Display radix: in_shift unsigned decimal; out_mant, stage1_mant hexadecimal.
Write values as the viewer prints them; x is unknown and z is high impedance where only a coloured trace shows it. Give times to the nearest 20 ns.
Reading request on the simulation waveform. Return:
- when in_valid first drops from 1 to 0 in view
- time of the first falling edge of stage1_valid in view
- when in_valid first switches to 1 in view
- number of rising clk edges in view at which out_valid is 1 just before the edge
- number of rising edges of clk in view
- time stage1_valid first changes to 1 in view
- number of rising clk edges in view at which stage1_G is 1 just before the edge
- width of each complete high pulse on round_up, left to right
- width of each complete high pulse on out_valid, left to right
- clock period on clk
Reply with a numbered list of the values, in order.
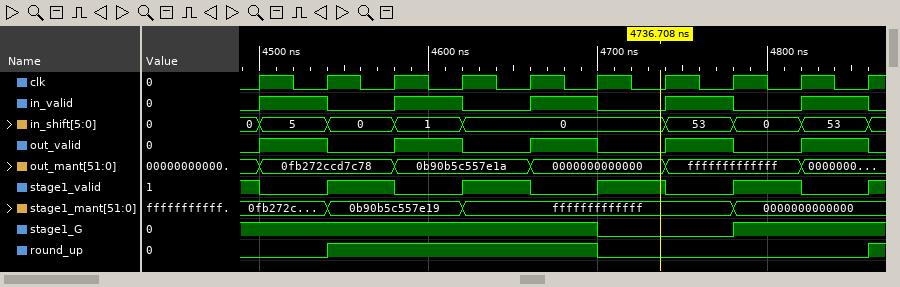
1. 4540 ns
2. 4500 ns
3. 4500 ns
4. 5
5. 10
6. 4540 ns
7. 8
8. 160 ns
9. 40 ns, 40 ns, 40 ns, 40 ns, 40 ns
10. 40 ns
